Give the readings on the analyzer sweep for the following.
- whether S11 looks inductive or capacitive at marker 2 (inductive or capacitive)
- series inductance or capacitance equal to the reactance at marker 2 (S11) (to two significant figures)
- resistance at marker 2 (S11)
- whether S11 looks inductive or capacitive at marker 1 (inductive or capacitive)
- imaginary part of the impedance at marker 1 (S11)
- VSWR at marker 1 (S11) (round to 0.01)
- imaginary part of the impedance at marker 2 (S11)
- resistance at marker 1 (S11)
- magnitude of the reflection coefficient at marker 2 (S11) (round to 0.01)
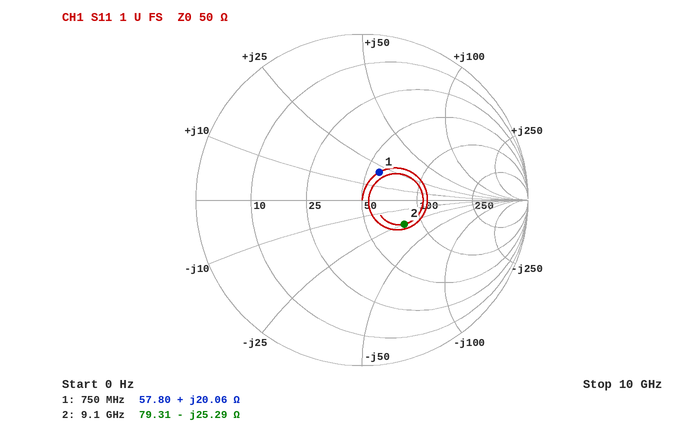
capacitive
690 fF
79.31 Ω
inductive
+20.06 Ω
1.49
-25.29 Ω
57.80 Ω
0.29
